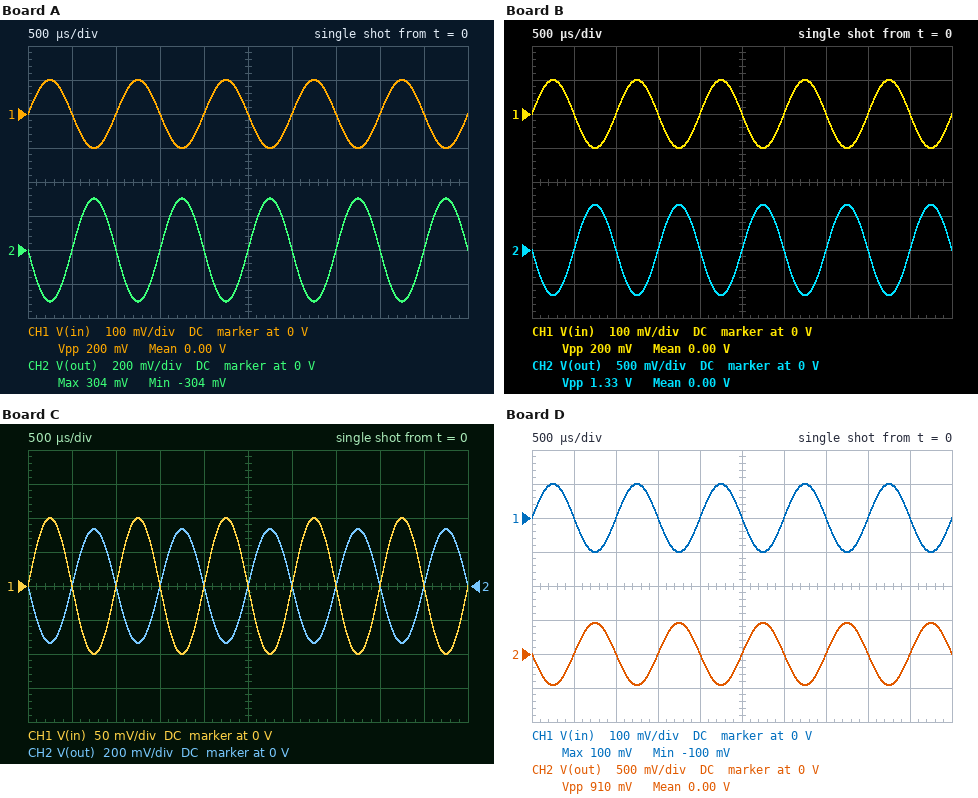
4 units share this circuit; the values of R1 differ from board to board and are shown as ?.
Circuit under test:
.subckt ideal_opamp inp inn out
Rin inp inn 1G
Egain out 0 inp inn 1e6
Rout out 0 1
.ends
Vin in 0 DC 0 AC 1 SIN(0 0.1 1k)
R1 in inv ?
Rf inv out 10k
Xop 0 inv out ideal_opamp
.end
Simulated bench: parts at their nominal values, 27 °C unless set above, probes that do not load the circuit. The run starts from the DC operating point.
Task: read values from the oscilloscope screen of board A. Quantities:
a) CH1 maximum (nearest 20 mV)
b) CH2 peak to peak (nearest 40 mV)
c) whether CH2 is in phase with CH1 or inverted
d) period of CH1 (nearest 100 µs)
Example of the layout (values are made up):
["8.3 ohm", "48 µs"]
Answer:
["100 mV", "600 mV", "inverted", "1.0 ms"]
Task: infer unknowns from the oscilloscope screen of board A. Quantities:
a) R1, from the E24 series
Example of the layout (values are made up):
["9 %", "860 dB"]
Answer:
["3.3 kΩ"]
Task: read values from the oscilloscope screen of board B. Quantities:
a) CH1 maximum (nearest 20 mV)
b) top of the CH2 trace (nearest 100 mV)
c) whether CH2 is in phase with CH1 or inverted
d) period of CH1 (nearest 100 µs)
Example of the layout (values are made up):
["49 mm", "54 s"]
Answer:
["100 mV", "700 mV", "inverted", "1.0 ms"]
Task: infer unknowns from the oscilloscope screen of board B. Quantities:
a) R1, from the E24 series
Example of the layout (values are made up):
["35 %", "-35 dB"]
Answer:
["1.5 kΩ"]
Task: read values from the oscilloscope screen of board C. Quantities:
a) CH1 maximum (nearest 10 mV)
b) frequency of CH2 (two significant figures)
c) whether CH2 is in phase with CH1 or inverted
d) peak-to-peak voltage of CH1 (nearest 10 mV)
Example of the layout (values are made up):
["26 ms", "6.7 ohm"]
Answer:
["100 mV", "1.0 kHz", "inverted", "200 mV"]
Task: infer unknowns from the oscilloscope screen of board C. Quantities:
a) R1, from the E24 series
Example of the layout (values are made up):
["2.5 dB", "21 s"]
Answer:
["3 kΩ"]
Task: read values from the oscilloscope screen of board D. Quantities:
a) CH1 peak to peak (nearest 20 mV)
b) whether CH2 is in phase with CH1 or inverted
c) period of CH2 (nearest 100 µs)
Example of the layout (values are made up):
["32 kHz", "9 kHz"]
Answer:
["200 mV", "inverted", "1.0 ms"]
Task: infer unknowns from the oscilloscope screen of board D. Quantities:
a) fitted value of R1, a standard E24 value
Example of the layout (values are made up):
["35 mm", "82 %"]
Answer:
["2.2 kΩ"]
